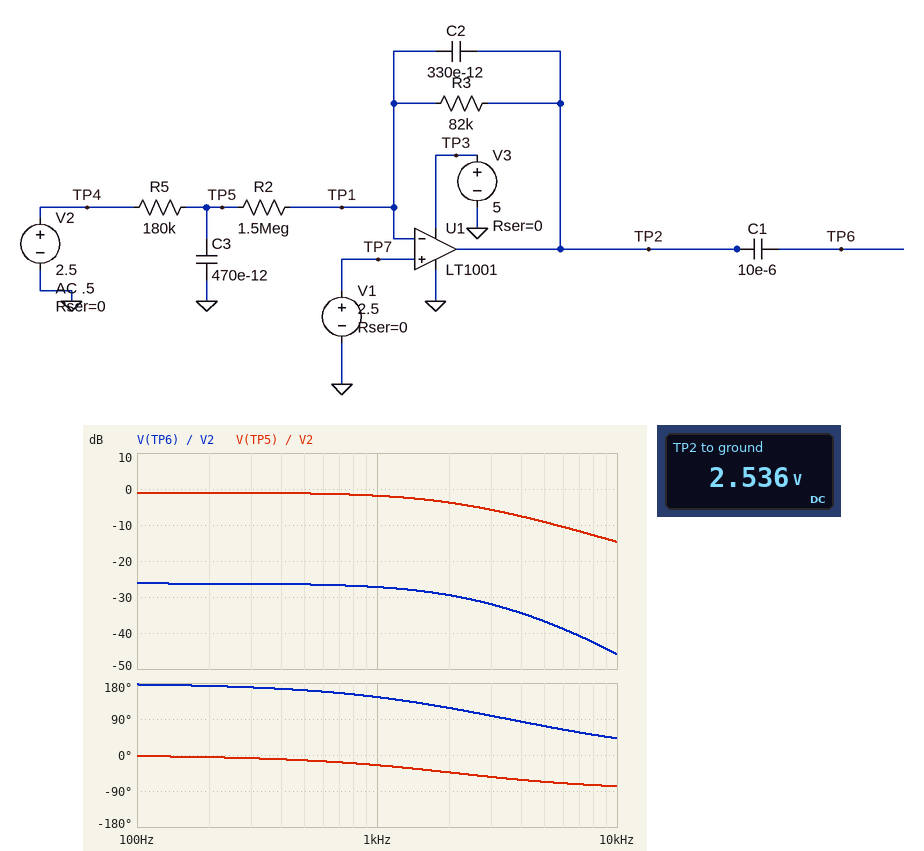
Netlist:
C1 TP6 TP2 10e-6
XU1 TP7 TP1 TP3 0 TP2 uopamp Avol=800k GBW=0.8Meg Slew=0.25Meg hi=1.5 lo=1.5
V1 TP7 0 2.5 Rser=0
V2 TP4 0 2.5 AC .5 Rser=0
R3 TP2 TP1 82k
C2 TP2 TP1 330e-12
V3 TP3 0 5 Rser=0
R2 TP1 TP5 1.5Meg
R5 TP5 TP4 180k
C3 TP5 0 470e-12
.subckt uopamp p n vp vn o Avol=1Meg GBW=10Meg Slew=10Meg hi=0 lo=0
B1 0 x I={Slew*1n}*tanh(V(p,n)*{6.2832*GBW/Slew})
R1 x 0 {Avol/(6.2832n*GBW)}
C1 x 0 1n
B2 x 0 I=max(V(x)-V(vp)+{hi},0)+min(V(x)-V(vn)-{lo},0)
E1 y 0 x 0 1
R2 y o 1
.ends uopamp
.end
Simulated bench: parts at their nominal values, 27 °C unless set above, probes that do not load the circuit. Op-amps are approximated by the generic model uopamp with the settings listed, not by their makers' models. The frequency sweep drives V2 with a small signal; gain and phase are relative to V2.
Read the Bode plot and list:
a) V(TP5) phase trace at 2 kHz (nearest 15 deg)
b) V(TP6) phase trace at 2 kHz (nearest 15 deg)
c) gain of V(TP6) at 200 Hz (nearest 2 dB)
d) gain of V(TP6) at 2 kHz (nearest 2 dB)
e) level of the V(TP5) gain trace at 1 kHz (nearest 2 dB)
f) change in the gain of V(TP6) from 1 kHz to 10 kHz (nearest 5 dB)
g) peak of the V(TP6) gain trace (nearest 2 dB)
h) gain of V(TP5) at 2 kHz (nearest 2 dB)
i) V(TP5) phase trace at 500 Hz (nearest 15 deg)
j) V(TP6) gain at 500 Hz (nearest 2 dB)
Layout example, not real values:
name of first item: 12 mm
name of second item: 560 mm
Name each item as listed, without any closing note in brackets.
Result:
V(TP5) phase trace at 2 kHz: -45 deg
V(TP6) phase trace at 2 kHz: 120 deg
gain of V(TP6) at 200 Hz: -26 dB
gain of V(TP6) at 2 kHz: -30 dB
level of the V(TP5) gain trace at 1 kHz: -2 dB
change in the gain of V(TP6) from 1 kHz to 10 kHz: -20 dB
peak of the V(TP6) gain trace: -26 dB
gain of V(TP5) at 2 kHz: -4 dB
V(TP5) phase trace at 500 Hz: -15 deg
V(TP6) gain at 500 Hz: -26 dB
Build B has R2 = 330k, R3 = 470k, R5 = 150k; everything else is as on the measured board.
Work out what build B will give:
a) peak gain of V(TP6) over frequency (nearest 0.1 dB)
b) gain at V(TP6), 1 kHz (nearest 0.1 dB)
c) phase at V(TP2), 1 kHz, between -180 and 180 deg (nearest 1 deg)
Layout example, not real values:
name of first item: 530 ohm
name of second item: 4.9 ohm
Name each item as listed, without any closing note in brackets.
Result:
peak gain of V(TP6) over frequency: -0.2 dB
gain at V(TP6), 1 kHz: -3.5 dB
phase at V(TP2), 1 kHz, between -180 and 180 deg: 119 deg
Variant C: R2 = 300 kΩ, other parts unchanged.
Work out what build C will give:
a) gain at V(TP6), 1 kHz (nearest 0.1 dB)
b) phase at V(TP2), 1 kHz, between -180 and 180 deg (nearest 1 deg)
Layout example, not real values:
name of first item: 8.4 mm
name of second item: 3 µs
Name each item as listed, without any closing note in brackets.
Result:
gain at V(TP6), 1 kHz: -15.9 dB
phase at V(TP2), 1 kHz, between -180 and 180 deg: 152 deg
